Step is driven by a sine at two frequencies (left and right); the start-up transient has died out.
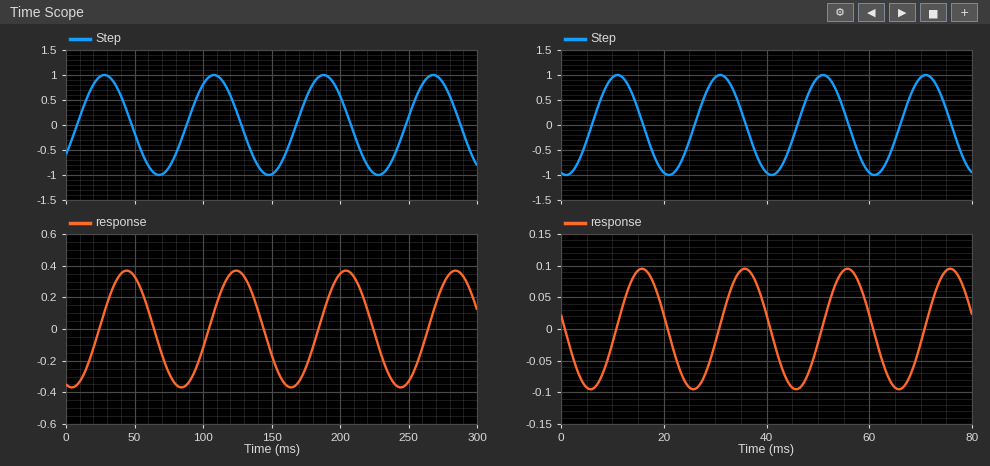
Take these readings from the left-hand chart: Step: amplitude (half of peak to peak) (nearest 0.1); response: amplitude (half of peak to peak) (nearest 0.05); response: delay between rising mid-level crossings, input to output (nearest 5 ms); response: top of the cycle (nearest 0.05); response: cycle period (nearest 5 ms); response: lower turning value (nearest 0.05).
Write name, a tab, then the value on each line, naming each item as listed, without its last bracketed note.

Step: amplitude (half of peak to peak)	1.0
response: amplitude (half of peak to peak)	0.35
response: delay between rising mid-level crossings, input to output	15 ms
response: top of the cycle	0.35
response: cycle period	80 ms
response: lower turning value	-0.35
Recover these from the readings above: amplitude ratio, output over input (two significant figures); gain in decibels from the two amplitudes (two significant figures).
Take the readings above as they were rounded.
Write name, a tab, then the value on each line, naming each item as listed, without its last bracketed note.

amplitude ratio, output over input	0.35
gain in decibels from the two amplitudes	-9.1 dB
